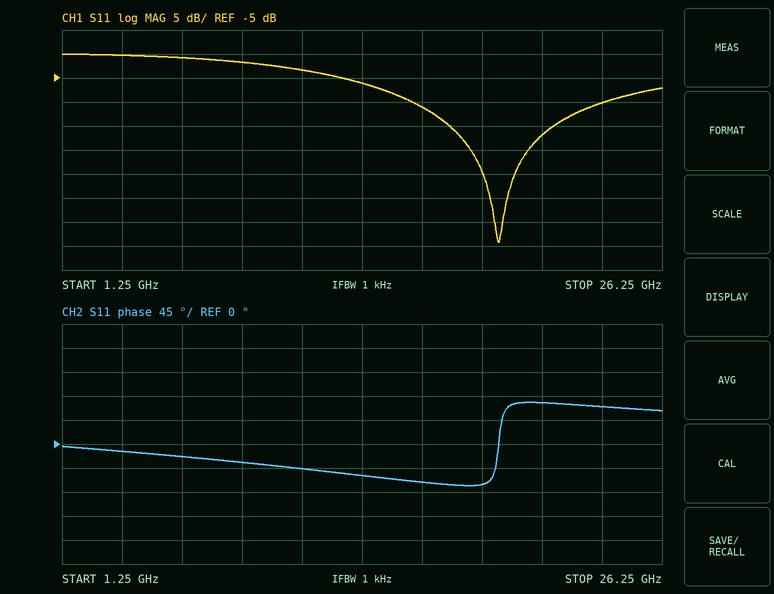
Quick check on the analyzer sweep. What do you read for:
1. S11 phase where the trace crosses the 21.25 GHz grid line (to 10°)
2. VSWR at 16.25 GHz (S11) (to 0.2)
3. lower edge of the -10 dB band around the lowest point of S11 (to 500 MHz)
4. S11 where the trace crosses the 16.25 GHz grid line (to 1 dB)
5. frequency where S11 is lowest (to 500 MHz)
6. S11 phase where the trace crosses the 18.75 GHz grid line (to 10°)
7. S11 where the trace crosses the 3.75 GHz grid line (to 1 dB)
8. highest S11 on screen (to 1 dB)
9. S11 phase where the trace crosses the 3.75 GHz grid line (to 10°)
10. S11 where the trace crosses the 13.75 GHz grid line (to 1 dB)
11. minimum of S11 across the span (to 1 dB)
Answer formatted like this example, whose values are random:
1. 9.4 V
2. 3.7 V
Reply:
1. 80°
2. 1.8
3. 16.0 GHz
4. -11 dB
5. 19.5 GHz
6. -80°
7. 0 dB
8. 0 dB
9. -10°
10. -6 dB
11. -39 dB
